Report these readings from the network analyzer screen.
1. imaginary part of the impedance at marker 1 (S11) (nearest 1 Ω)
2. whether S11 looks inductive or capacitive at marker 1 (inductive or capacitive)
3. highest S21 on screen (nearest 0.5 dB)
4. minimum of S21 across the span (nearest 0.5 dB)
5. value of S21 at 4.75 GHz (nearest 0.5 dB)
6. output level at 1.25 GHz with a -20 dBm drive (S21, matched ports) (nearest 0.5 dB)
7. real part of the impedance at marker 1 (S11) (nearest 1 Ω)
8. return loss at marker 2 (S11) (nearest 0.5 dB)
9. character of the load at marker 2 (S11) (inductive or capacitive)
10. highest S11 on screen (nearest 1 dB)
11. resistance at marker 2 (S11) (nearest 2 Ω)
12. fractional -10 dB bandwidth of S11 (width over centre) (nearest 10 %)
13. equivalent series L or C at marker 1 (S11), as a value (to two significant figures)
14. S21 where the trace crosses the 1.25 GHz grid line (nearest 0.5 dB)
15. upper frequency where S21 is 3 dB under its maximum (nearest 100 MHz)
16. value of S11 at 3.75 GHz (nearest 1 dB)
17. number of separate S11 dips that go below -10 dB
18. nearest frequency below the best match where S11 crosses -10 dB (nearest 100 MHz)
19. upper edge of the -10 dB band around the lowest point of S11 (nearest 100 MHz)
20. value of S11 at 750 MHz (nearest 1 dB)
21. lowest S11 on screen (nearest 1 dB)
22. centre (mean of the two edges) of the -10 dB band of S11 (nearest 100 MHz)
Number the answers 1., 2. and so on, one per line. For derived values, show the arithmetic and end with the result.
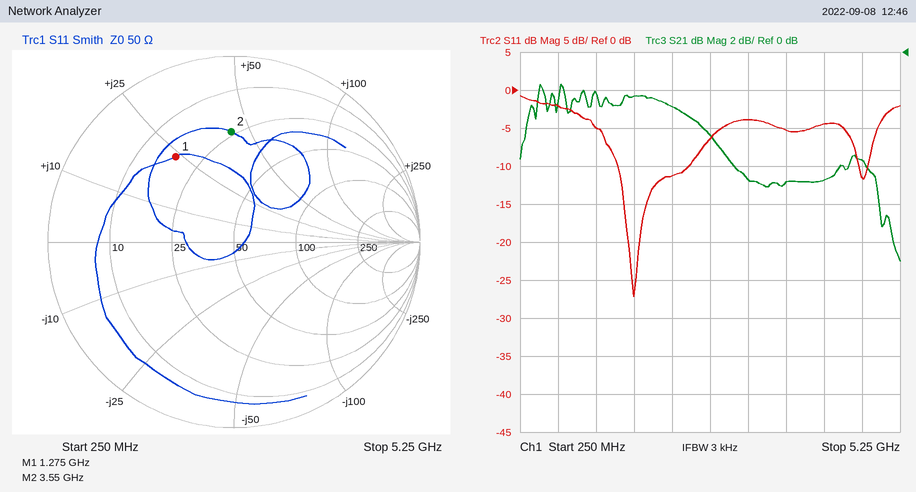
1. +24 Ω
2. inductive
3. -1.5 dB
4. -11.0 dB
5. -5.5 dB
6. -20 dBm + (-2.0 dB) = -22.0 dBm
7. 18 Ω
8. 4.5 dB
9. inductive
10. -1 dB
11. 24 Ω
12. 1 GHz / 2 GHz ≈ 50 %
13. L = 24 Ω/(2π × 1.275 GHz) ≈ 3.0 nH
14. -2.0 dB
15. 2.8 GHz
16. -5 dB
17. 2
18. 1.5 GHz
19. 2.5 GHz
20. -2 dB
21. -27 dB
22. 2.0 GHz
